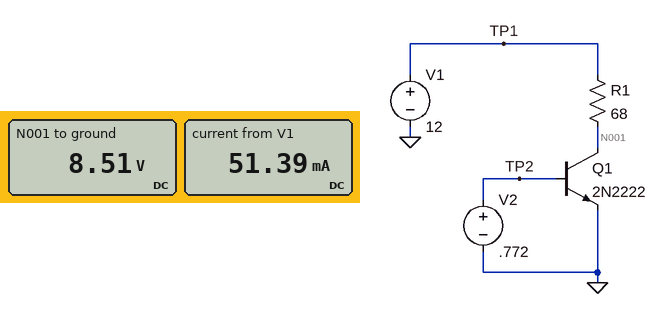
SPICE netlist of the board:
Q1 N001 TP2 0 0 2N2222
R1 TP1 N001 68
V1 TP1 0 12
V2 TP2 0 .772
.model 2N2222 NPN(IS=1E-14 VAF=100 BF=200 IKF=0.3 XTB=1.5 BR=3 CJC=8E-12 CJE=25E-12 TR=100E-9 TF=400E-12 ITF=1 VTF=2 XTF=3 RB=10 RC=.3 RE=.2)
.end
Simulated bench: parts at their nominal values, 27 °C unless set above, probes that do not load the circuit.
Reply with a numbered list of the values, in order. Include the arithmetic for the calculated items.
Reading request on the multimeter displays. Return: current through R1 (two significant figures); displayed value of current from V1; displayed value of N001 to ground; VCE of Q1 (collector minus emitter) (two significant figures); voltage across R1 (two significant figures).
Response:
1. (12 V - 8.51 V) / 68 Ω = 51 mA
2. 51.39 mA
3. 8.51 V
4. 8.51 V = 8.5 V
5. 12 V - 8.51 V = 3.5 V
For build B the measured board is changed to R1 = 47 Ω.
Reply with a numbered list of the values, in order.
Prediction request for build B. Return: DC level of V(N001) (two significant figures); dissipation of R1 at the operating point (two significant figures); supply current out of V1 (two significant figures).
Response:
1. 9.6 V
2. 130 mW
3. 52 mA
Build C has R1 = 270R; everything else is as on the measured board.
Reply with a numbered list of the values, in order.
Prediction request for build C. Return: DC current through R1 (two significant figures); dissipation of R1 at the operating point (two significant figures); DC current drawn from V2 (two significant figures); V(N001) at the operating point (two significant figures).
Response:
1. 44 mA
2. 520 mW
3. 570 µA
4. 130 mV
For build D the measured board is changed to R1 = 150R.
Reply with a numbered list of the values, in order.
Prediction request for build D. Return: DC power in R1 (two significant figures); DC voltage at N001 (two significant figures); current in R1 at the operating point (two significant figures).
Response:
1. 370 mW
2. 4.5 V
3. 50 mA
